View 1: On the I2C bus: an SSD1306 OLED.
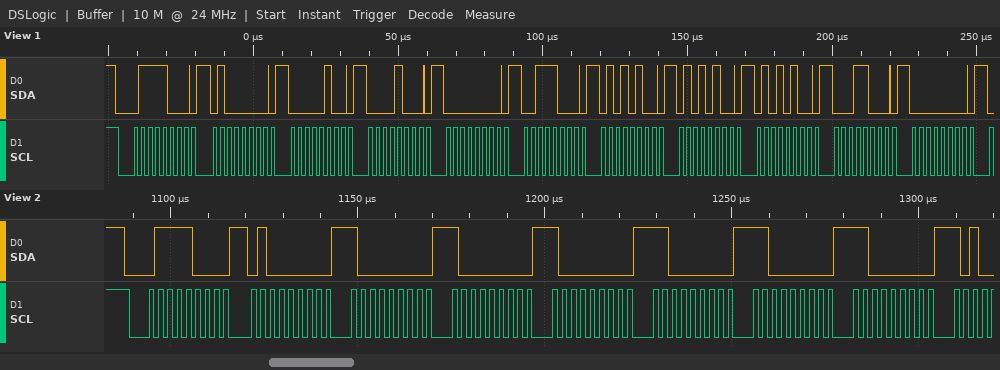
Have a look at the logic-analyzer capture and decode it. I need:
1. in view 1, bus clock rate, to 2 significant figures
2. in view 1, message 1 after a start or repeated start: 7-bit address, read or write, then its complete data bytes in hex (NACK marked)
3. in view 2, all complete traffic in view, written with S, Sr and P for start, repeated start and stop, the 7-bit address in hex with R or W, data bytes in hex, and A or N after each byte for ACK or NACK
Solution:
400 kHz
0x3C write: 40 04 08 00 38 54 54 54 18 00
S 3CW A 40 A 80 A 80 A 80 A C0 A C0 A C0 A
